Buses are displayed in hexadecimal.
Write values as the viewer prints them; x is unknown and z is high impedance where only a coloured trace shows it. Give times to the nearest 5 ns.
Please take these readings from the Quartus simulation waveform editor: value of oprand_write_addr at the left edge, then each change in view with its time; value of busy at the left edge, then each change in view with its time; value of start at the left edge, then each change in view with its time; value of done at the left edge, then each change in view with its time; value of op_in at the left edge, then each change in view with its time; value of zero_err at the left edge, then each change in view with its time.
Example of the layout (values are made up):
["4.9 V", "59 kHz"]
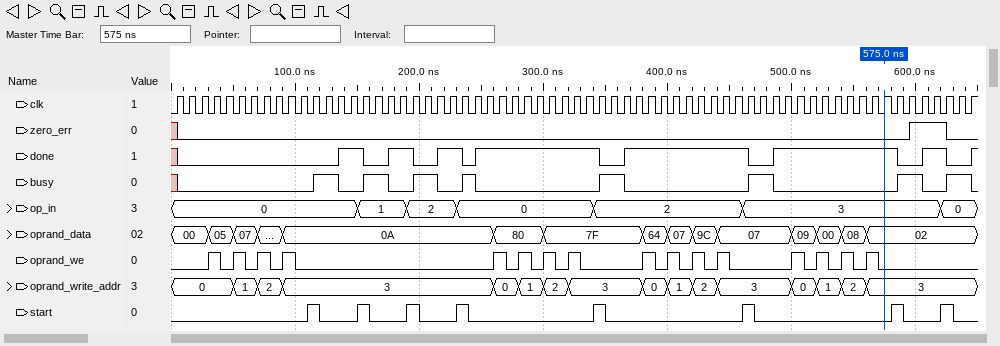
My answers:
["0, 1 at 50 ns, 2 at 70 ns, 3 at 90 ns, 0 at 260 ns, 1 at 280 ns, 2 at 300 ns, 3 at 320 ns, 0 at 380 ns, 1 at 400 ns, 2 at 420 ns, 3 at 440 ns, 0 at 500 ns, 1 at 520 ns, 2 at 540 ns, 3 at 560 ns", "x, 0 at 5 ns, 1 at 115 ns, 0 at 135 ns, 1 at 155 ns, 0 at 175 ns, 1 at 195 ns, 0 at 215 ns, 1 at 235 ns, 0 at 245 ns, 1 at 345 ns, 0 at 365 ns, 1 at 465 ns, 0 at 485 ns, 1 at 585 ns, 0 at 605 ns, 1 at 625 ns, 0 at 645 ns", "0, 1 at 110 ns, 0 at 120 ns, 1 at 150 ns, 0 at 160 ns, 1 at 190 ns, 0 at 200 ns, 1 at 230 ns, 0 at 240 ns, 1 at 340 ns, 0 at 350 ns, 1 at 460 ns, 0 at 470 ns, 1 at 580 ns, 0 at 590 ns, 1 at 620 ns, 0 at 630 ns", "x, 0 at 5 ns, 1 at 135 ns, 0 at 155 ns, 1 at 175 ns, 0 at 195 ns, 1 at 215 ns, 0 at 235 ns, 1 at 245 ns, 0 at 345 ns, 1 at 365 ns, 0 at 465 ns, 1 at 485 ns, 0 at 585 ns, 1 at 605 ns, 0 at 625 ns, 1 at 645 ns", "0, 1 at 150 ns, 2 at 190 ns, 0 at 230 ns, 2 at 340 ns, 3 at 460 ns, 0 at 620 ns", "x, 0 at 5 ns, 1 at 595 ns, 0 at 625 ns"]
